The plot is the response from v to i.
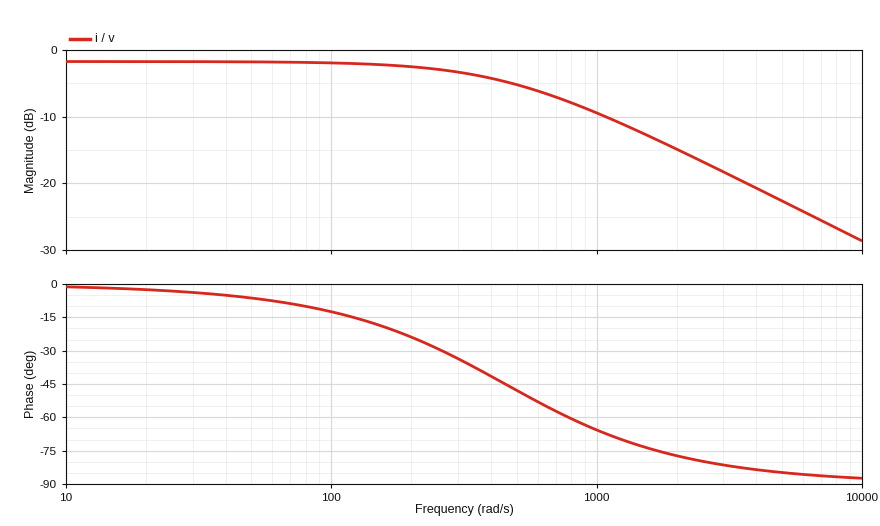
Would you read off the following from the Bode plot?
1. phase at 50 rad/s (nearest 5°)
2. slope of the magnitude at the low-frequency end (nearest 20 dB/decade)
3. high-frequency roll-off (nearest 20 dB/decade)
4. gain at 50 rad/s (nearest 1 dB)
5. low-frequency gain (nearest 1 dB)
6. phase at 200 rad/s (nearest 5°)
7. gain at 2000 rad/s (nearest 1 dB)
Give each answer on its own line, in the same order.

-5°
0 dB/decade
-20 dB/decade
-2 dB
-2 dB
-25°
-15 dB
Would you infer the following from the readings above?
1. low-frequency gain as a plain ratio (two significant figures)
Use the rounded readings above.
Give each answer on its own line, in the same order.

0.79
